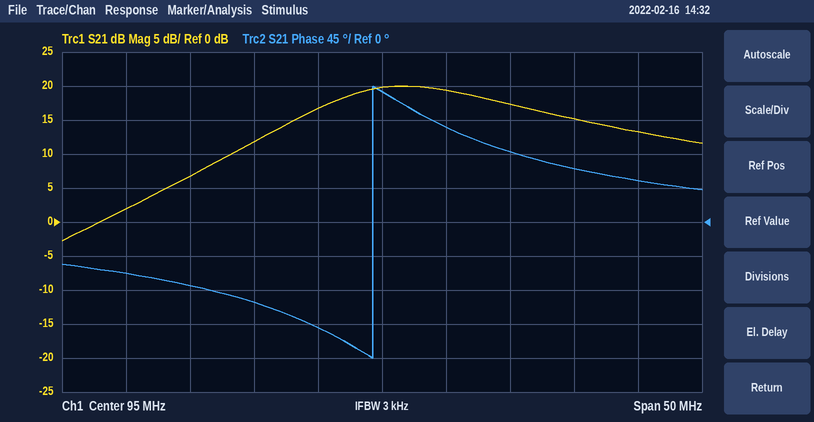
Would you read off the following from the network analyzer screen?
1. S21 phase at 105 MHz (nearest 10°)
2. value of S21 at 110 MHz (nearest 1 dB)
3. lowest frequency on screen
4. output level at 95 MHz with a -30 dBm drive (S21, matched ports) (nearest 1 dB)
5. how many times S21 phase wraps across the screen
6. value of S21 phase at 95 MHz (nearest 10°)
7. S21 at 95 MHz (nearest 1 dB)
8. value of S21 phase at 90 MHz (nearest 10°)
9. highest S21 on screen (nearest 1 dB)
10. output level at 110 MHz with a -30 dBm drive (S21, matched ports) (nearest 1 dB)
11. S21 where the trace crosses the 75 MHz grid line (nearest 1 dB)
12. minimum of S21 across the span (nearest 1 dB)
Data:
90°
15 dB
70 MHz
-10 dBm
1
170°
20 dB
-140°
20 dB
-15 dBm
2 dB
-3 dB
